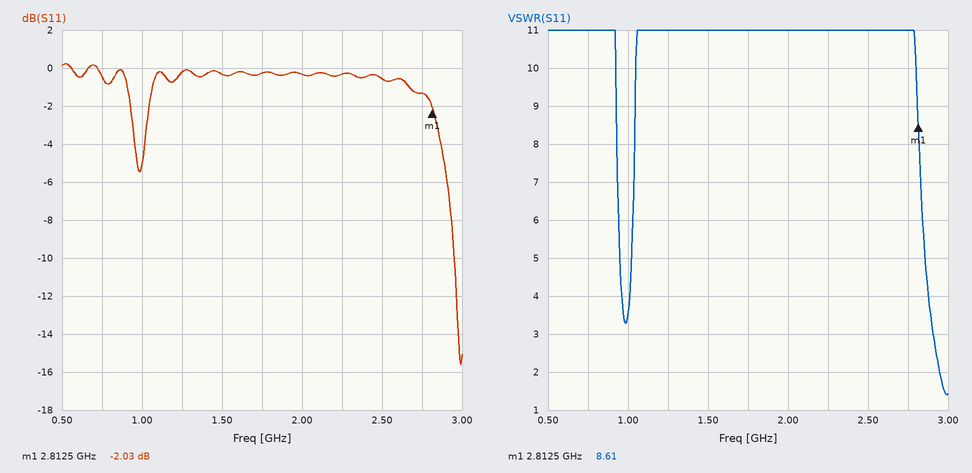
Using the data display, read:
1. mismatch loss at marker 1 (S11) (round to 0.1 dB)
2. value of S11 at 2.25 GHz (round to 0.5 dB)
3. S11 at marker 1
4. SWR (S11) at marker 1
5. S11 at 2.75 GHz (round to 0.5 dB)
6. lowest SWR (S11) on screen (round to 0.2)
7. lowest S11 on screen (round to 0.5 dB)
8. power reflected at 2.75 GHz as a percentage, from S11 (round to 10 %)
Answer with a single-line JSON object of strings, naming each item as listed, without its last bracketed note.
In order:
{"mismatch loss at marker 1 (S11)": "4.3 dB", "value of S11 at 2.25 GHz": "-0.5 dB", "S11 at marker 1": "-2.03 dB", "SWR (S11) at marker 1": "8.61", "S11 at 2.75 GHz": "-1.5 dB", "lowest SWR (S11) on screen": "1.4", "lowest S11 on screen": "-15.5 dB", "power reflected at 2.75 GHz as a percentage, from S11": "70 %"}
